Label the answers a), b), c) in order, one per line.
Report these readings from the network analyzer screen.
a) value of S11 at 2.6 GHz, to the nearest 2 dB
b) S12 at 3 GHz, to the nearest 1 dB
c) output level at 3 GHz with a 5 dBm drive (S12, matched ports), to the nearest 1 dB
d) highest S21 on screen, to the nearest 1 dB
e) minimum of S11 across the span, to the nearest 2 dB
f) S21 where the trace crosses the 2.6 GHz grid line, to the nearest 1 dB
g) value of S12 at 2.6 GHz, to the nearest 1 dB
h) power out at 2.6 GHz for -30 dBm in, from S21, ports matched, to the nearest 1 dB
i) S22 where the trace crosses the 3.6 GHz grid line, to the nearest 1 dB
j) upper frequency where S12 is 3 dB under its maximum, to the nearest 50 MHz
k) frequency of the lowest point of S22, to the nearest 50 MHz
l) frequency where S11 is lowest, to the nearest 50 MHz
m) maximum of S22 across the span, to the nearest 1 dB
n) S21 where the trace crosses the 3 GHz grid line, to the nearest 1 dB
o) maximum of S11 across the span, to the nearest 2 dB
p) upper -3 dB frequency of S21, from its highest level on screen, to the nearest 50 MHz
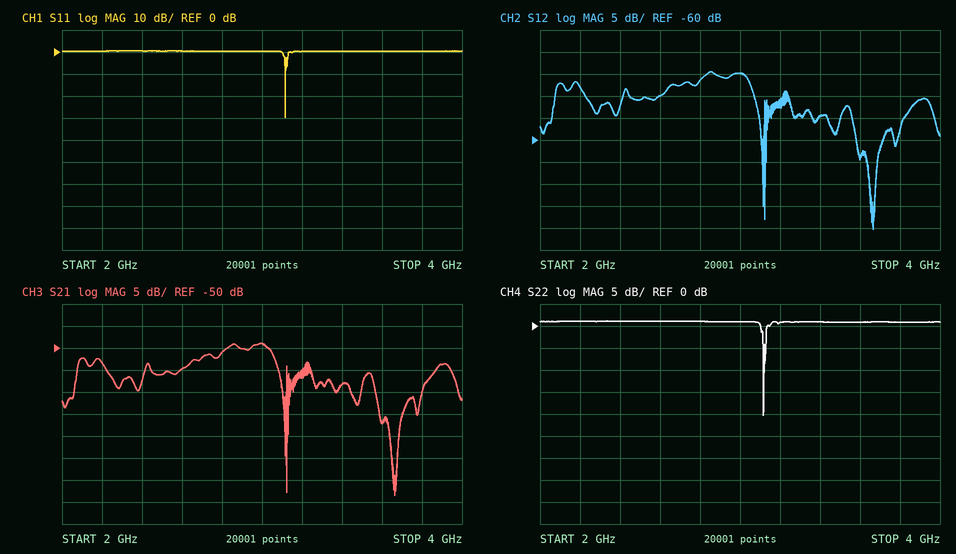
a) 0 dB
b) -45 dB
c) -40 dBm
d) -49 dB
e) -30 dB
f) -55 dB
g) -50 dB
h) -85 dBm
i) 1 dB
j) 3.05 GHz
k) 3.10 GHz
l) 3.10 GHz
m) 1 dB
n) -49 dB
o) 0 dB
p) 3.05 GHz
